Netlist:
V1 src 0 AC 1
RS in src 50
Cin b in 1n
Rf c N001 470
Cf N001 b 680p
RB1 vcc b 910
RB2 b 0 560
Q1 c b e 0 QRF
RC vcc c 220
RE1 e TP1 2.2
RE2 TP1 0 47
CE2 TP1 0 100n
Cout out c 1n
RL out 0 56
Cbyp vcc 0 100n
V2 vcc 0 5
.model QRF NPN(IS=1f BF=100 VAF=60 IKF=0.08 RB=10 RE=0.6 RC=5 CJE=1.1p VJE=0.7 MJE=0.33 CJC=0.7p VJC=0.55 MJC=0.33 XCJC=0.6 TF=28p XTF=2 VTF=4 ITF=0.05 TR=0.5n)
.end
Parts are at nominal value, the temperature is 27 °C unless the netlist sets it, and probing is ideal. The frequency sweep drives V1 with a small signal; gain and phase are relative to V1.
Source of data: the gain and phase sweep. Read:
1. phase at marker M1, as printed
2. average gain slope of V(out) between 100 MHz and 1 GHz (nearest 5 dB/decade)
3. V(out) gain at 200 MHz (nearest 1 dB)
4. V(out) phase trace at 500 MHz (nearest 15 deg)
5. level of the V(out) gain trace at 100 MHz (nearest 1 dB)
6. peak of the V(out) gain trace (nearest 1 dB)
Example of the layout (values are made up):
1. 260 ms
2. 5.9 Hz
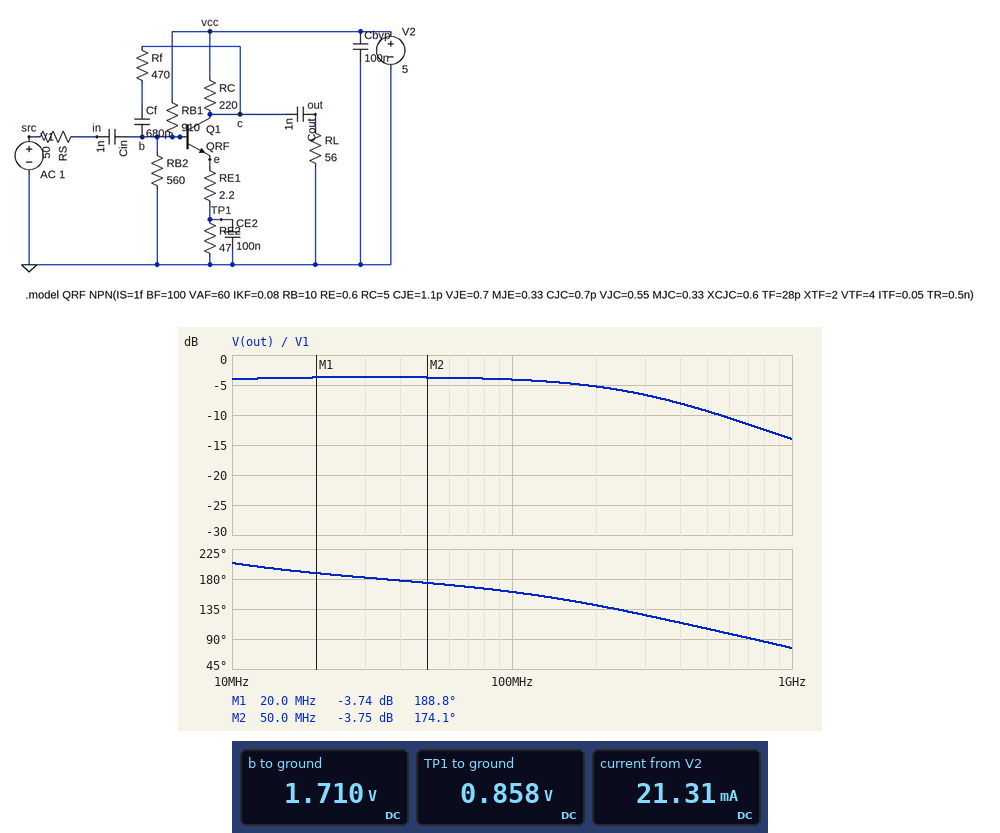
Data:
1. 188.8 deg
2. -10 dB/decade
3. -5 dB
4. 105 deg
5. -4 dB
6. -4 dB
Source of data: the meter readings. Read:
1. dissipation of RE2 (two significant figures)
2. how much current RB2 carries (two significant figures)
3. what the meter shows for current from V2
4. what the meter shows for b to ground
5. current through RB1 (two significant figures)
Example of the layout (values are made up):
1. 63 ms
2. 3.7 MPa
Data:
1. 16 mW
2. 3.1 mA
3. 21.31 mA
4. 1.710 V
5. 3.6 mA
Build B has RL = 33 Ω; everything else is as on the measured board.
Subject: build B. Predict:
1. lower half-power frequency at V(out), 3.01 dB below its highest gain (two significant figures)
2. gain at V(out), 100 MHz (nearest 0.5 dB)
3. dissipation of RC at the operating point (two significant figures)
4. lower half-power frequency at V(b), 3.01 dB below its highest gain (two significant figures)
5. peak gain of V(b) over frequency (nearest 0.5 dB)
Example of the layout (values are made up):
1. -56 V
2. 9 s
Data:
1. 4.4 MHz
2. -5.0 dB
3. 69 mW
4. 2.9 MHz
5. -11.0 dB
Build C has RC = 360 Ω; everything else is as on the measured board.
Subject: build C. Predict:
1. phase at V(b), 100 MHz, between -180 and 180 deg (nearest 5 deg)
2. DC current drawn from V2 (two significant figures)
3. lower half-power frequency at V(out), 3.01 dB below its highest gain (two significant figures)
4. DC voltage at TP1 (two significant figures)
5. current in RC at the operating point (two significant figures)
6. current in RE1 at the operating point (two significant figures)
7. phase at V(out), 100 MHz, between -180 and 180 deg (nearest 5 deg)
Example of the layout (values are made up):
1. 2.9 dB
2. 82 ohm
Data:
1. 0 deg
2. 16 mA
3. 3.7 MHz
4. 610 mV
5. 12 mA
6. 13 mA
7. 155 deg
